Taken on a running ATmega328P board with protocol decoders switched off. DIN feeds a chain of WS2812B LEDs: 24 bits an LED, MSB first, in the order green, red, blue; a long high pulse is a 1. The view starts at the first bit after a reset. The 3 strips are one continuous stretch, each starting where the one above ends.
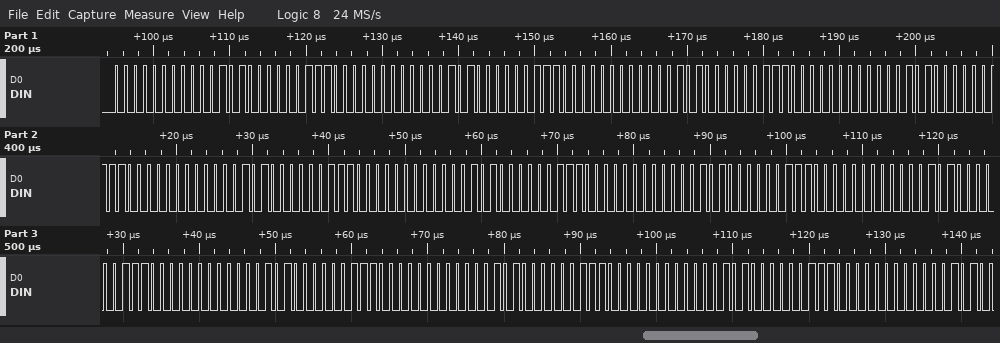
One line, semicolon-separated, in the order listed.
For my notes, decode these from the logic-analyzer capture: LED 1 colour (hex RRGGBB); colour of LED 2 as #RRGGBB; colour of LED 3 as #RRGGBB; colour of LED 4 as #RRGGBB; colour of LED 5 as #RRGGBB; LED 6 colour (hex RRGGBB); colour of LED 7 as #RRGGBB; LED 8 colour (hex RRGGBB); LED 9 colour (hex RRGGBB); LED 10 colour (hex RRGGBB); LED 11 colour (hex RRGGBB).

#14000E; #14000E; #14000E; #14000E; #14000E; #14000E; #14000E; #14000E; #14000E; #14000E; #14000E
